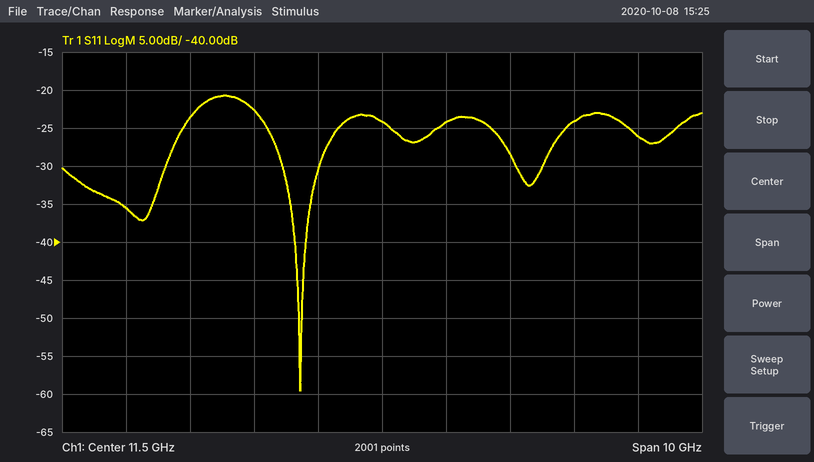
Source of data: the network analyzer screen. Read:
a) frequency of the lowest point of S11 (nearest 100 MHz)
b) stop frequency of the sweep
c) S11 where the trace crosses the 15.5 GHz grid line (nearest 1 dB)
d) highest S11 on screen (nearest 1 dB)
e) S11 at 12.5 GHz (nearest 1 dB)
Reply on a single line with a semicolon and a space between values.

10.2 GHz; 16.5 GHz; -26 dB; -21 dB; -24 dB
